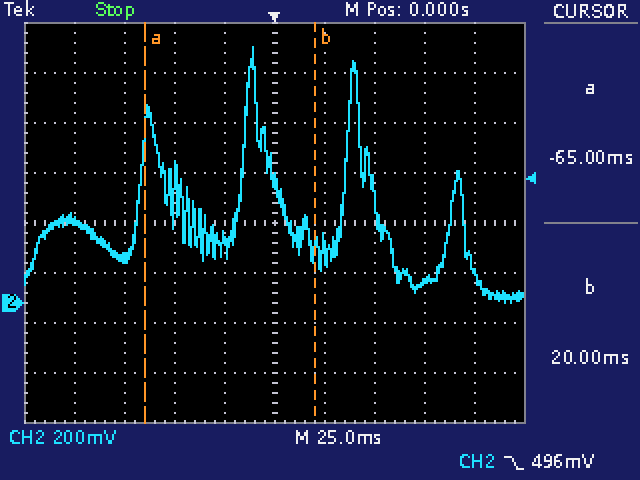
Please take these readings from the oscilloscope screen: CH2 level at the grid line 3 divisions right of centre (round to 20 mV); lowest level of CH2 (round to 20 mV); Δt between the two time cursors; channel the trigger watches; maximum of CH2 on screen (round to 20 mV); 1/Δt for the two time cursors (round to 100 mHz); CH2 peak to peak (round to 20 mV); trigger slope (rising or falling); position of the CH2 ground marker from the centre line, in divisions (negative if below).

80 mV
0 mV
85.0 ms
CH2
1.02 V
11.8 Hz
1.02 V
falling
-1.6 div
